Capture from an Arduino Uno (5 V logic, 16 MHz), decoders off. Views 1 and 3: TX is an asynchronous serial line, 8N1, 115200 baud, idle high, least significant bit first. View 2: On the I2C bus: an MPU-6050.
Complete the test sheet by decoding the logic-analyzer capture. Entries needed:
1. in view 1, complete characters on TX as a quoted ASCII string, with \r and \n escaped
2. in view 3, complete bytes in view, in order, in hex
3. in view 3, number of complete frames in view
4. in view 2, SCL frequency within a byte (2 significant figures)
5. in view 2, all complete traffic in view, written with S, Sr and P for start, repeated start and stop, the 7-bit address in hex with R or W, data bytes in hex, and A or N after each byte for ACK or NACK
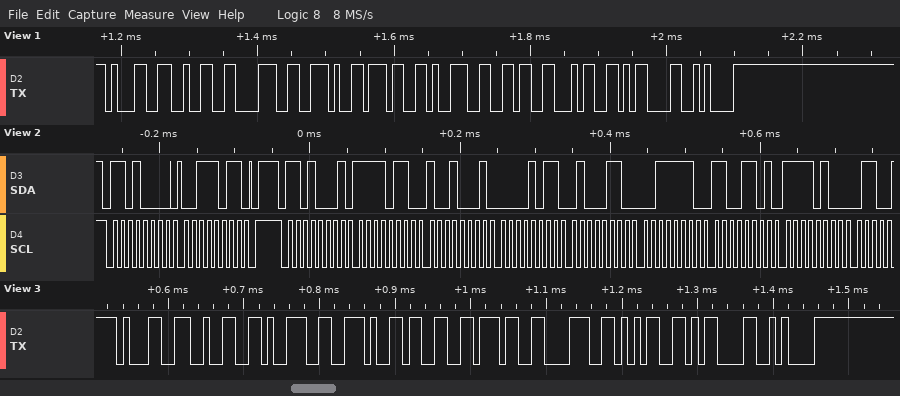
"128.7964\r\n"
0x31 0x32 0x39 0x2E 0x33 0x37 0x38 0x35 0x0D 0x0A
10
100 kHz
S 68W A 3B A P S 68R A F6 A 91 A 0B A 46 A 3E A CD A F4 A
